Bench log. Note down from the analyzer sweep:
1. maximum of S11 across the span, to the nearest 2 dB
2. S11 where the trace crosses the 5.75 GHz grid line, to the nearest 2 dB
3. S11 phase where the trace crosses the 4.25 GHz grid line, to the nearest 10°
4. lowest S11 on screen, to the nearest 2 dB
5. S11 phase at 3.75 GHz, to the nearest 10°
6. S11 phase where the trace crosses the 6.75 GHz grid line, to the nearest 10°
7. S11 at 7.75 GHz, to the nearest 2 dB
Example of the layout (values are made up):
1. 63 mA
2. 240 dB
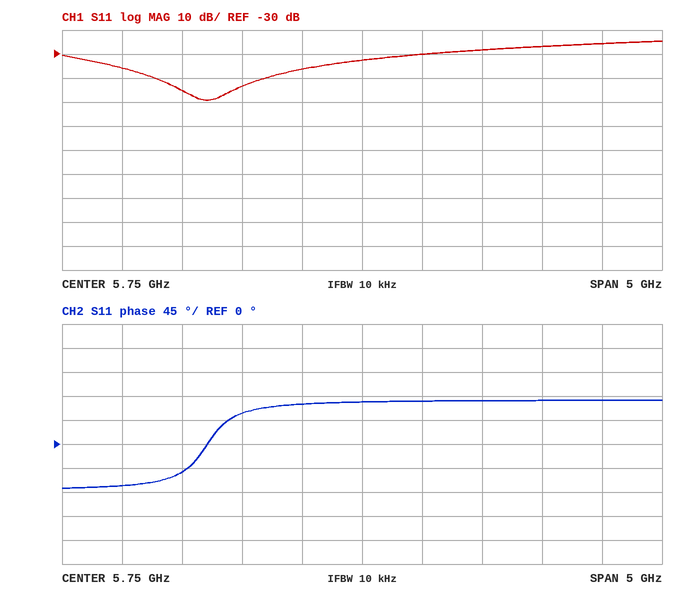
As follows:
1. -24 dB
2. -32 dB
3. -50°
4. -50 dB
5. -80°
6. 80°
7. -26 dB
